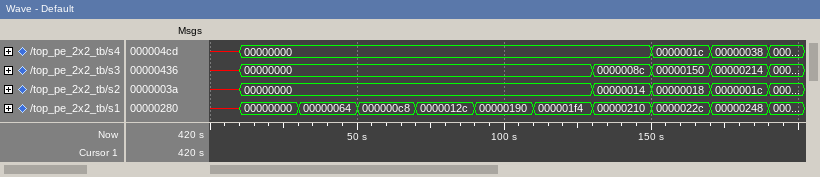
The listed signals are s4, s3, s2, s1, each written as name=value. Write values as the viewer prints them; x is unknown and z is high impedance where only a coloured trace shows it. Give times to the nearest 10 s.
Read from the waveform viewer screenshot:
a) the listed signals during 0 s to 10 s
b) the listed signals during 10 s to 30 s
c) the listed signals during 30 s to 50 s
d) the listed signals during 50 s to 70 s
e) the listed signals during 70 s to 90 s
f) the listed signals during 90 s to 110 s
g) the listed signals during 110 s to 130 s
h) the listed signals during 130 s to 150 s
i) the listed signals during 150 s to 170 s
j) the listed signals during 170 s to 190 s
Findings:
s4=x, s3=x, s2=x, s1=x
s4=00000000, s3=00000000, s2=00000000, s1=00000000
s4=00000000, s3=00000000, s2=00000000, s1=00000064
s4=00000000, s3=00000000, s2=00000000, s1=000000c8
s4=00000000, s3=00000000, s2=00000000, s1=0000012c
s4=00000000, s3=00000000, s2=00000000, s1=00000190
s4=00000000, s3=00000000, s2=00000000, s1=000001f4
s4=00000000, s3=0000008c, s2=00000014, s1=00000210
s4=0000001c, s3=00000150, s2=00000018, s1=0000022c
s4=00000038, s3=00000214, s2=0000001c, s1=00000248
